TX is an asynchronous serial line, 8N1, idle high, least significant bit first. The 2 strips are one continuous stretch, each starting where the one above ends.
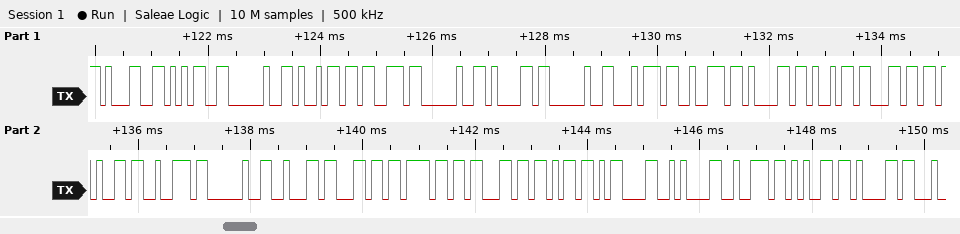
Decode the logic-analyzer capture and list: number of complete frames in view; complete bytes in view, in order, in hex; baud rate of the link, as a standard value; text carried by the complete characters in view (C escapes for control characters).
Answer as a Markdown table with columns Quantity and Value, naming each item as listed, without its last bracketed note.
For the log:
| Quantity | Value |
|---|---|
| number of complete frames in view | 26 |
| complete bytes in view, in order, in hex | 31 35 20 69 73 20 61 20 74 72 61 69 6C 65 72 20 62 6C 6F 63 6B 0D 0A 72 65 61 |
| baud rate of the link, as a standard value | 9600 baud |
| text carried by the complete characters in view | "15 is a trailer block\r\nrea" |
